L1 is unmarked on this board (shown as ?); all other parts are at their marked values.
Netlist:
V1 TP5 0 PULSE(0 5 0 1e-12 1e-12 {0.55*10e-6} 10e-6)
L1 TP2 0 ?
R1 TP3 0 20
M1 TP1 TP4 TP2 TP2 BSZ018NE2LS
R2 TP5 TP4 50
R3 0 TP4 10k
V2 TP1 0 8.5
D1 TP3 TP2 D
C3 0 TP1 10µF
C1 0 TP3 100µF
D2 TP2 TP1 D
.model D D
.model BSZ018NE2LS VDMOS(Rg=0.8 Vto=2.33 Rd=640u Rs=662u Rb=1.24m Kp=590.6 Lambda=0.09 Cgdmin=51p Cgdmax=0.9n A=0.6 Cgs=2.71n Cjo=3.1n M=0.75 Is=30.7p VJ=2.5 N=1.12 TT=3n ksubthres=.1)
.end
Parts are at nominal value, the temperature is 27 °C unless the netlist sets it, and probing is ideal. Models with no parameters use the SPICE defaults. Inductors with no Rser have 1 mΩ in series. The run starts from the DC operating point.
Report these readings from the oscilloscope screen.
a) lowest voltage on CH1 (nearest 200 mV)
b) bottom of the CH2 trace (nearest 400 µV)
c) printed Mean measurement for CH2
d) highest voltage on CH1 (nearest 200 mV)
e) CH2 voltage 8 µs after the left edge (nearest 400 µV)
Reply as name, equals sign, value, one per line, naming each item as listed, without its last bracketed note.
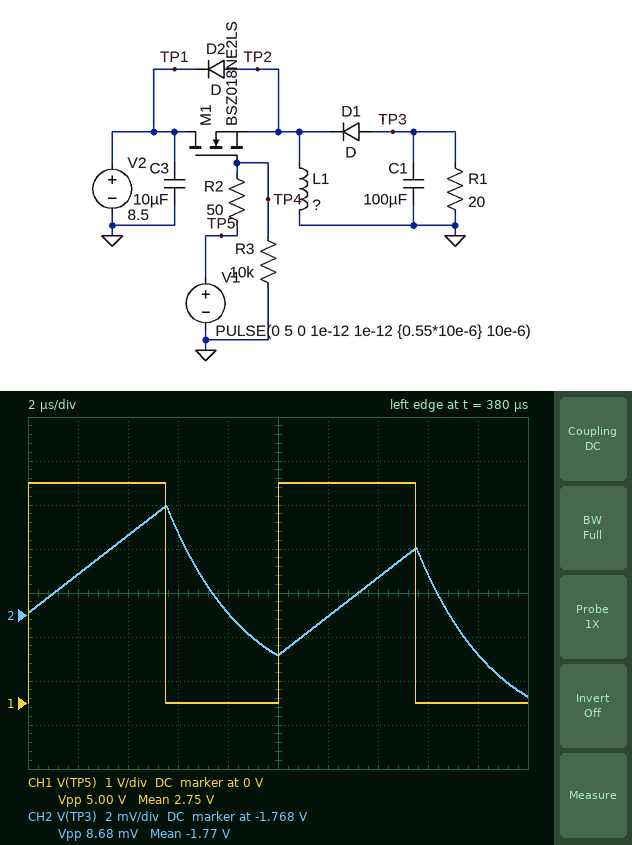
lowest voltage on CH1 = 0 V
bottom of the CH2 trace = -1.7716 V
printed Mean measurement for CH2 = -1.77 V
highest voltage on CH1 = 5.0 V
CH2 voltage 8 µs after the left edge = -1.7680 V
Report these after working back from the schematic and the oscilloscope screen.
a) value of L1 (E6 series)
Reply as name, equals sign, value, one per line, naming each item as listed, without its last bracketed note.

value of L1 = 3.3 µH
